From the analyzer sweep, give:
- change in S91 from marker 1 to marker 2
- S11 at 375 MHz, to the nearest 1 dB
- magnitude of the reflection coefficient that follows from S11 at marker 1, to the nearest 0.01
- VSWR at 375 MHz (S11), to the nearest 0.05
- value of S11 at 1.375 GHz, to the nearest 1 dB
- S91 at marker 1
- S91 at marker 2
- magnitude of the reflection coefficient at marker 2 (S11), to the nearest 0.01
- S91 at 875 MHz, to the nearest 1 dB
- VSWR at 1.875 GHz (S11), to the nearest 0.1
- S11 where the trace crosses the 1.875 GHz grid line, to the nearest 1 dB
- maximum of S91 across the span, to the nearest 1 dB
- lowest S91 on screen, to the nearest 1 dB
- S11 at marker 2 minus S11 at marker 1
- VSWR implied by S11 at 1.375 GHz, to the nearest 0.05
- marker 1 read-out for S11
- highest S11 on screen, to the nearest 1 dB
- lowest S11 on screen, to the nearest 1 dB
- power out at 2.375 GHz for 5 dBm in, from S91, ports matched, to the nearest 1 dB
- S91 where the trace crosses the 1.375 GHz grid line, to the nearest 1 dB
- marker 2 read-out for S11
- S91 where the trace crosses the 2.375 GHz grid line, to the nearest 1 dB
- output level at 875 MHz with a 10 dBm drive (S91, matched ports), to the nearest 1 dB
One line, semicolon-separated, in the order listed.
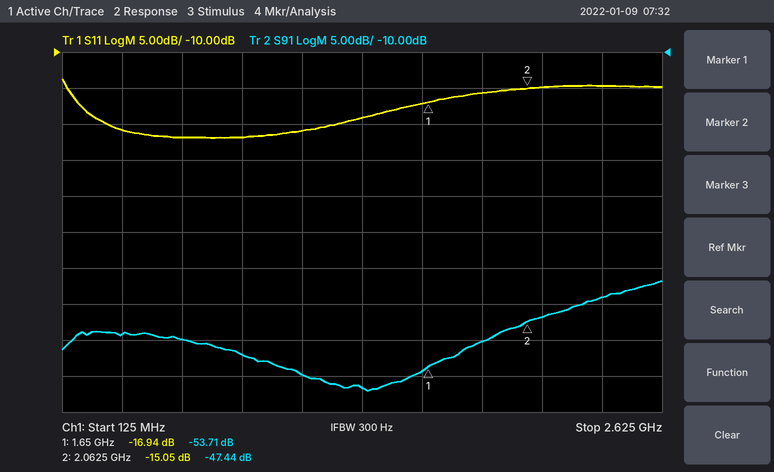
6.27 dB; -21 dB; 0.14; 1.20; -19 dB; -53.71 dB; -47.44 dB; 0.18; -52 dB; 1.4; -16 dB; -42 dB; -57 dB; 1.89 dB; 1.25; -16.94 dB; -14 dB; -22 dB; -39 dBm; -57 dB; -15.05 dB; -44 dB; -42 dBm
